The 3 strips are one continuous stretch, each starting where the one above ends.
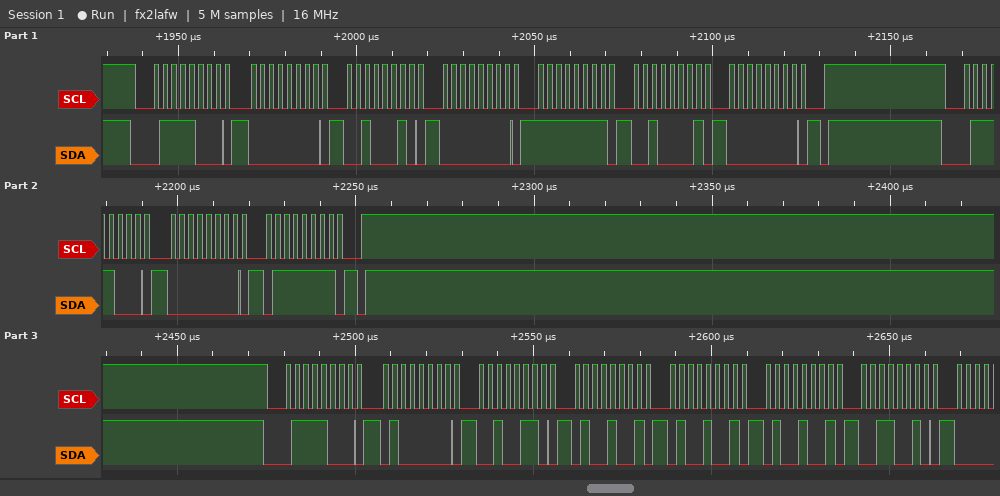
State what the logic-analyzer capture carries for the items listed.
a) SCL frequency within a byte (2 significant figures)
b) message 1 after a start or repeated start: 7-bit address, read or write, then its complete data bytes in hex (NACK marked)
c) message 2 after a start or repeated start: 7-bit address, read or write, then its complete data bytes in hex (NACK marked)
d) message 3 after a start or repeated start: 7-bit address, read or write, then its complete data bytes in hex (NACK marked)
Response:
400 kHz
0x3C write: 00 22 00 FF 21 00
0x3C write: 00 7F
0x3C write: 40 26 49 49 49 32
